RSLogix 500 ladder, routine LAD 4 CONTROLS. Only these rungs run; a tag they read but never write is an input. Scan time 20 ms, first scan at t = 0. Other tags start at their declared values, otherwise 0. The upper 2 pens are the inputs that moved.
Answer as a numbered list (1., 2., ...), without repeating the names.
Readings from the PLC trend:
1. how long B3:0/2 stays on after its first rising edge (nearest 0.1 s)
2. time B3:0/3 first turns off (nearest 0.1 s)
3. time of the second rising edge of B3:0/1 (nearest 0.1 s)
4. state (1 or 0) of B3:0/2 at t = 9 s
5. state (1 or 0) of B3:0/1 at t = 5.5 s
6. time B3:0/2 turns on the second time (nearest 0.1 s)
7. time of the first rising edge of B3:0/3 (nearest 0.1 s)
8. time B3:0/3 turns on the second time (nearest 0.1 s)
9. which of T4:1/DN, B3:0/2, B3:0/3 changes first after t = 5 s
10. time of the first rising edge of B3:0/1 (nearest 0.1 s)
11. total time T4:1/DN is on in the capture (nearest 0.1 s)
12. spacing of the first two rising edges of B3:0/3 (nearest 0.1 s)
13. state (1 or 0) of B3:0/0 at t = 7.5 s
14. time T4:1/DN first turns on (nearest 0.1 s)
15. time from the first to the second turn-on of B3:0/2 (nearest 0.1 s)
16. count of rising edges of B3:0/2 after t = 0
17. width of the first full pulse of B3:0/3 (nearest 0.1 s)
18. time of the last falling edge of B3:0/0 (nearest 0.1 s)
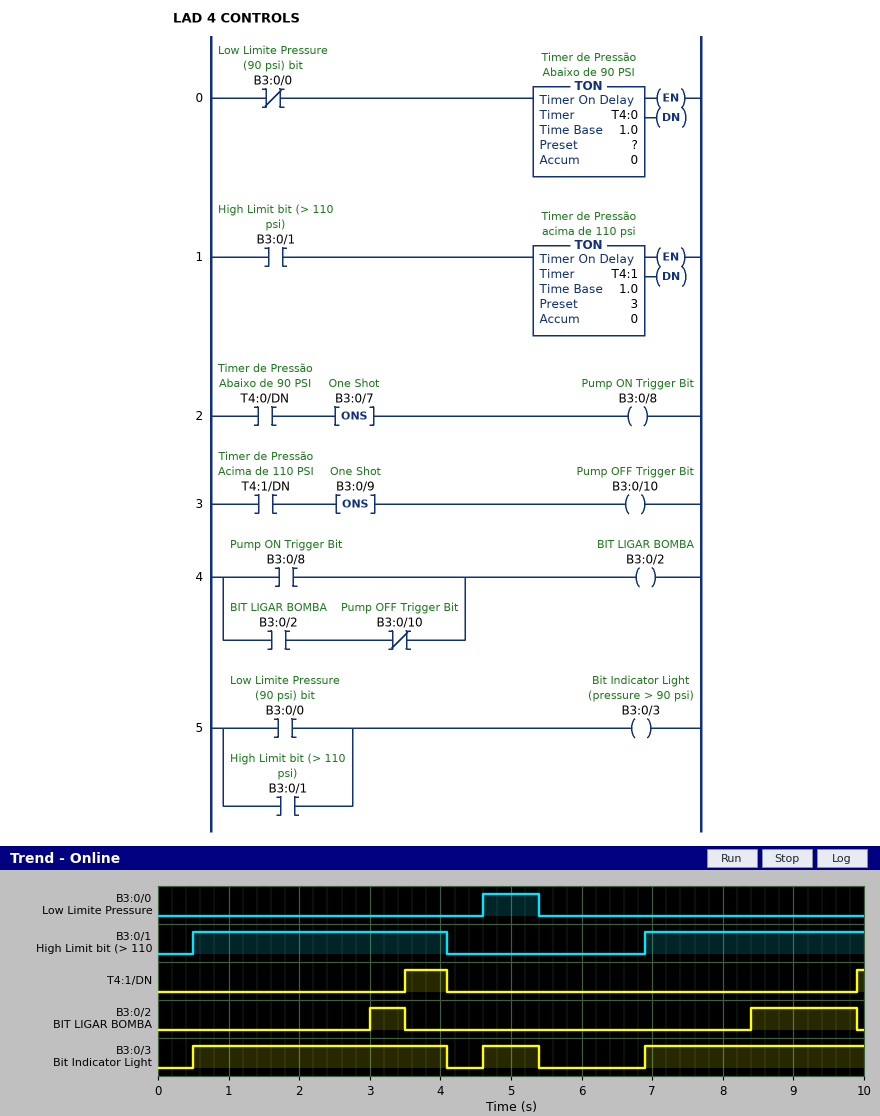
1. 0.5 s
2. 4.1 s
3. 6.9 s
4. 1
5. 0
6. 8.4 s
7. 0.5 s
8. 4.6 s
9. B3:0/3
10. 0.5 s
11. 0.7 s
12. 4.1 s
13. 0
14. 3.5 s
15. 5.4 s
16. 2
17. 3.6 s
18. 5.4 s
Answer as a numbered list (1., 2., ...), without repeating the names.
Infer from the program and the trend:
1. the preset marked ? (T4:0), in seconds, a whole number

1. 3 s
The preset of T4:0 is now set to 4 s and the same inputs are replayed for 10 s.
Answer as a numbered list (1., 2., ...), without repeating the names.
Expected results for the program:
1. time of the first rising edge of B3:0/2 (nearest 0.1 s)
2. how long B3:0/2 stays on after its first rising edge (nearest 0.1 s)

1. 4.0 s
2. 5.9 s
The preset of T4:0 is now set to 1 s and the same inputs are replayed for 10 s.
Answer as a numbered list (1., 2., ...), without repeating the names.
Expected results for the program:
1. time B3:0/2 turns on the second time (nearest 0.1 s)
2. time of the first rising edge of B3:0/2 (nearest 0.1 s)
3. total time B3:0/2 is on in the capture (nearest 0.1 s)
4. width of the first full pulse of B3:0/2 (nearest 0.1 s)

1. 6.4 s
2. 1.0 s
3. 6.0 s
4. 2.5 s
